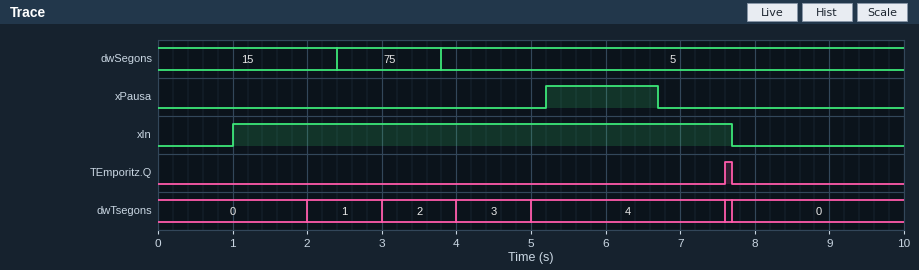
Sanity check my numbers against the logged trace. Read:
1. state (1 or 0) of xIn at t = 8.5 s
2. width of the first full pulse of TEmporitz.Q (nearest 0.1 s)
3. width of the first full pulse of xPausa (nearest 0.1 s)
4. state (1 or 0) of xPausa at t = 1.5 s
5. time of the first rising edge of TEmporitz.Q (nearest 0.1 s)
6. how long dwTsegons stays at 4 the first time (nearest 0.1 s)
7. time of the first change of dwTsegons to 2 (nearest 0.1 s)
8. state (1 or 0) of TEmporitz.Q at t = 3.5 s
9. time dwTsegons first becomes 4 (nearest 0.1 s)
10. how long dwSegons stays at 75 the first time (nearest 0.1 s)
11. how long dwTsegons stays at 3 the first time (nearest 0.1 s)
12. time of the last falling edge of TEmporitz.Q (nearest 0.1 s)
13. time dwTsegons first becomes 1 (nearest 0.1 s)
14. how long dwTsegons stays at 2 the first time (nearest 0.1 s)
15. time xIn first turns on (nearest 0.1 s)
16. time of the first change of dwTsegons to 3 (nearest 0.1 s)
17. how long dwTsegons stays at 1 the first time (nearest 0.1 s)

0
0.1 s
1.5 s
0
7.6 s
2.6 s
3.0 s
0
5.0 s
1.4 s
1.0 s
7.7 s
2.0 s
1.0 s
1.0 s
4.0 s
1.0 s
